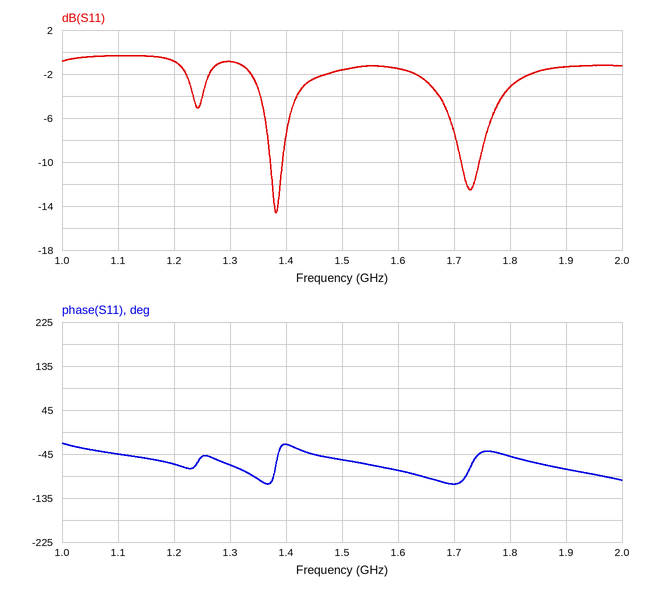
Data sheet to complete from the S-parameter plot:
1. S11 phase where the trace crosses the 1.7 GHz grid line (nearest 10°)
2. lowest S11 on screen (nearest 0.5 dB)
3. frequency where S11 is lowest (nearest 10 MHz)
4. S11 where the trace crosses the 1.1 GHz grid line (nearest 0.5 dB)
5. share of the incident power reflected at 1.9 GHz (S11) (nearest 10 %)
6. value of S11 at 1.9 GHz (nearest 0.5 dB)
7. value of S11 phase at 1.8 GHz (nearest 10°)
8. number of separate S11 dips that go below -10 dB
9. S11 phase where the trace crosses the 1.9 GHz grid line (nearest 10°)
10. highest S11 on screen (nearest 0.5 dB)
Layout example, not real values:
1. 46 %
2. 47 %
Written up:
1. -110°
2. -14.5 dB
3. 1.38 GHz
4. -0.5 dB
5. 70 %
6. -1.5 dB
7. -50°
8. 2
9. -80°
10. -0.5 dB
